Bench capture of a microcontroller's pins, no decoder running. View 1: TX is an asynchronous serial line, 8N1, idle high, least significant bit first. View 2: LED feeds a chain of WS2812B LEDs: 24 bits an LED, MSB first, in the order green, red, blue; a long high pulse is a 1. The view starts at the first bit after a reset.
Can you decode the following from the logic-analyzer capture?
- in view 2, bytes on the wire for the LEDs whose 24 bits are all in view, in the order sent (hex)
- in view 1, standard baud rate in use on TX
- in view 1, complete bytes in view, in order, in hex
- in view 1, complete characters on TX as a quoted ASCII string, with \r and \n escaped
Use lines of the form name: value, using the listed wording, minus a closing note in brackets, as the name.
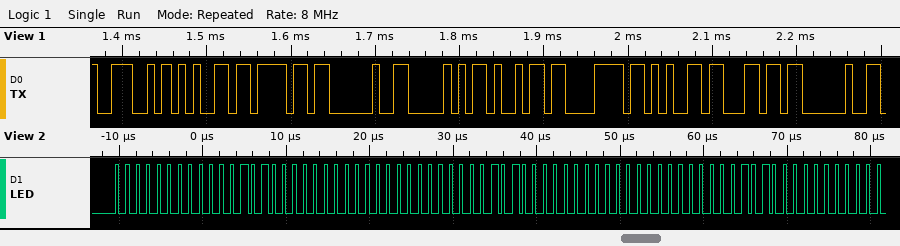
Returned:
in view 2, bytes on the wire for the LEDs whose 24 bits are all in view, in the order sent: 00 0A 00 00 0A 00 00 0A 00
in view 1, standard baud rate in use on TX: 115200 baud
in view 1, complete bytes in view, in order, in hex: 0x4E 0x65 0x6F 0x20 0x50 0x69 0x78 0x65 0x6C 0x20
in view 1, complete characters on TX as a quoted ASCII string, with \r and \n escaped: "Neo Pixel "
